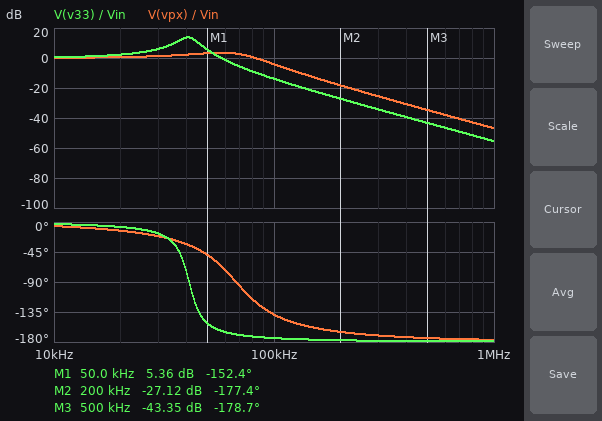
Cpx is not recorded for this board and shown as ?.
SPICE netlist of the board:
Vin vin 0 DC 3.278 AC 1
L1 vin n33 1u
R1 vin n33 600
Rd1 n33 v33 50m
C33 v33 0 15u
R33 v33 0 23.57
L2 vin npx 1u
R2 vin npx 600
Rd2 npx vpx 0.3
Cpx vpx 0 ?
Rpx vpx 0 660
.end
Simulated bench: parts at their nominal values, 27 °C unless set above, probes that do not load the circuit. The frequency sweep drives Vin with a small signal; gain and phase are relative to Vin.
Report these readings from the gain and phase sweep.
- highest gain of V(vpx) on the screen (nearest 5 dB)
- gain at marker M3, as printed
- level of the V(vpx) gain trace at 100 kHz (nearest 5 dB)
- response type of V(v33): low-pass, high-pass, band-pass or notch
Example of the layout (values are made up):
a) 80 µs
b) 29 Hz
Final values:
a) 5 dB
b) -43.35 dB
c) -5 dB
d) low-pass
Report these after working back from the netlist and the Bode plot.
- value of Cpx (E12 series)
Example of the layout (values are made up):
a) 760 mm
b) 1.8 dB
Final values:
a) 5.6 µF
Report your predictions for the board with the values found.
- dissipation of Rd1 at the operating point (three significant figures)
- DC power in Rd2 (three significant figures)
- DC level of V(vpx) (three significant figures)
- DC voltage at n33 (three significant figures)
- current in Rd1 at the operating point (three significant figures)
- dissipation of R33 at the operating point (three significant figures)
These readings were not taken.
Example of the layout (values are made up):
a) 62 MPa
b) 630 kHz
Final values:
a) 963 µW
b) 7.39 µW
c) 3.28 V
d) 3.28 V
e) 139 mA
f) 454 mW
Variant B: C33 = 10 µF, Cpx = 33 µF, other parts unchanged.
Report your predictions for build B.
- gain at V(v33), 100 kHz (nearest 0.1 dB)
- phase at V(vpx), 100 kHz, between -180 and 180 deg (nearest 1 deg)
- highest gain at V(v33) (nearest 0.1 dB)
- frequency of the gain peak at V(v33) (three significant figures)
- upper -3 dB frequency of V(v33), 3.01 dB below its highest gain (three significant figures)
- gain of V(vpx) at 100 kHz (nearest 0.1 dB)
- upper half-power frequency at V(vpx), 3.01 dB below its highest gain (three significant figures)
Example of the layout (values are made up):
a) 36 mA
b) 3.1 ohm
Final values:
a) -9.4 dB
b) -153 deg
c) 15.3 dB
d) 50.0 kHz
e) 54.2 kHz
f) -22.6 dB
g) 21.9 kHz
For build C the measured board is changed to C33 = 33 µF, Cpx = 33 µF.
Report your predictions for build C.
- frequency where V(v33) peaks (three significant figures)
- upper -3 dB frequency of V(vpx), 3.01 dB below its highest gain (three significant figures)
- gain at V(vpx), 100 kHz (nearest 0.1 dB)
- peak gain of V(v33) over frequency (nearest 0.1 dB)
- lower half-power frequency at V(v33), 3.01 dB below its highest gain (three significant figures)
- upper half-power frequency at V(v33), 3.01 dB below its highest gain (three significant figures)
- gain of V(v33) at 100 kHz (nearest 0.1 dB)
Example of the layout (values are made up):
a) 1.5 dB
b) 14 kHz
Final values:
a) 27.1 kHz
b) 21.9 kHz
c) -22.6 dB
d) 10.7 dB
e) 22.6 kHz
f) 31.0 kHz
g) -21.6 dB
